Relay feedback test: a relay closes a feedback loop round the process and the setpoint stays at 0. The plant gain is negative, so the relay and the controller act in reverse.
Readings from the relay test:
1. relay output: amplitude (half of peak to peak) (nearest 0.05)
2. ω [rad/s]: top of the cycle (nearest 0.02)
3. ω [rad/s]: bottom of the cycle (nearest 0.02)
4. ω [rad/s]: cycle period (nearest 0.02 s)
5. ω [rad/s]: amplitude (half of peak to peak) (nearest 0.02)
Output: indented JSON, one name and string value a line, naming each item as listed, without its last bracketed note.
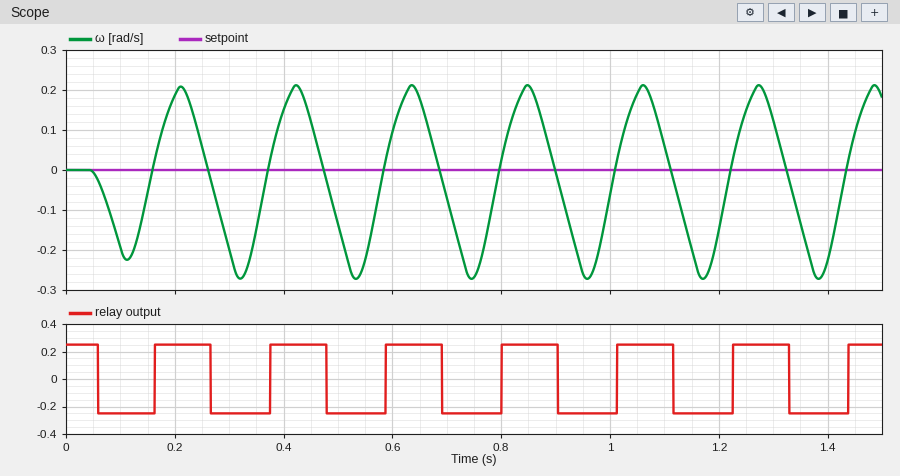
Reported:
{
  "relay output: amplitude (half of peak to peak)": "0.25",
  "ω [rad/s]: top of the cycle": "0.22",
  "ω [rad/s]: bottom of the cycle": "-0.28",
  "ω [rad/s]: cycle period": "0.22 s",
  "ω [rad/s]: amplitude (half of peak to peak)": "0.24"
}
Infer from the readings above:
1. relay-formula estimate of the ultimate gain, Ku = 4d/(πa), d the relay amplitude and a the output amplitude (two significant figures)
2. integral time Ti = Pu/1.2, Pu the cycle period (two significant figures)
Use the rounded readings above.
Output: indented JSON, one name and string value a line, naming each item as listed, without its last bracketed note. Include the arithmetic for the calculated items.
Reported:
{
  "relay-formula estimate of the ultimate gain, Ku = 4d/(πa), d the relay amplitude and a the output amplitude": "4 × 0.25 / (π × 0.24) = 1.3",
  "integral time Ti = Pu/1.2, Pu the cycle period": "0.22 / 1.2 = 0.18 s"
}
